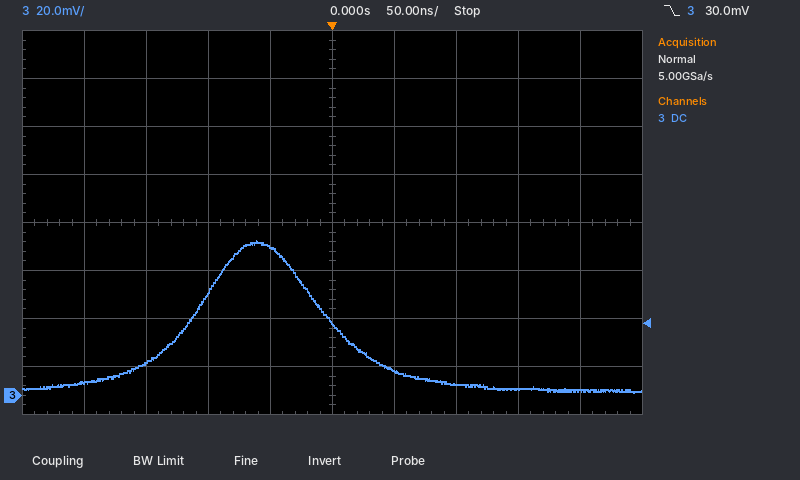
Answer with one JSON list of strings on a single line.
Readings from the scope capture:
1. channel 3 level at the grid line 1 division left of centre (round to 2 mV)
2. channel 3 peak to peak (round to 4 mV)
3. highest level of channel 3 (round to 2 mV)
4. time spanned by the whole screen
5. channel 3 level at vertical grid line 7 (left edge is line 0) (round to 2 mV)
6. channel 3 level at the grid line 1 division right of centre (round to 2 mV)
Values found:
["62 mV", "64 mV", "64 mV", "500 ns", "4 mV", "10 mV"]
